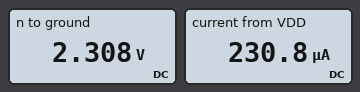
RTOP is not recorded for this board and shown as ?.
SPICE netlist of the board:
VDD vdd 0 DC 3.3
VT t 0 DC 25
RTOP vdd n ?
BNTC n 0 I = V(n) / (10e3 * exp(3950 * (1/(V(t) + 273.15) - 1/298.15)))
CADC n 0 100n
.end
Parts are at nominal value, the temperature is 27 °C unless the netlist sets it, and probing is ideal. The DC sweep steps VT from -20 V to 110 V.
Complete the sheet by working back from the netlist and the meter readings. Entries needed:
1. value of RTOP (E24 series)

4.3 kΩ
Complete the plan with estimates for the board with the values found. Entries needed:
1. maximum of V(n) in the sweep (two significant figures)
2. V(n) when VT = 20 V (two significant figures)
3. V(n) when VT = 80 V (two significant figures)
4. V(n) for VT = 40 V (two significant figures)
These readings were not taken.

3.2 V
2.5 V
750 mV
1.8 V
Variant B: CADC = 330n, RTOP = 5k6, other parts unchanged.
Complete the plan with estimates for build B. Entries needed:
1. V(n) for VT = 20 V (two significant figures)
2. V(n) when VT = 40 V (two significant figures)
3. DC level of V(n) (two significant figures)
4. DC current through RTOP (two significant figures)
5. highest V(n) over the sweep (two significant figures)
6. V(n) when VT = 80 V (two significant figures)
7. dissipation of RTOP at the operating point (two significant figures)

2.3 V
1.6 V
2.1 V
210 µA
3.1 V
610 mV
250 µW
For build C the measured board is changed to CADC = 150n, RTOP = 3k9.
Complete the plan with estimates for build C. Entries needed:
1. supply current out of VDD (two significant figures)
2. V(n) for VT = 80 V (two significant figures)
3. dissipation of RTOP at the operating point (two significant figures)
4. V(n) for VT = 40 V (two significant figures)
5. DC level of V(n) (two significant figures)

240 µA
810 mV
220 µW
1.9 V
2.4 V
